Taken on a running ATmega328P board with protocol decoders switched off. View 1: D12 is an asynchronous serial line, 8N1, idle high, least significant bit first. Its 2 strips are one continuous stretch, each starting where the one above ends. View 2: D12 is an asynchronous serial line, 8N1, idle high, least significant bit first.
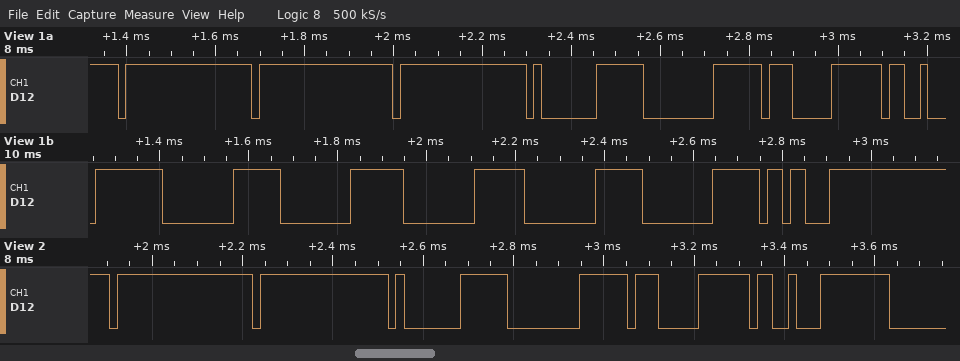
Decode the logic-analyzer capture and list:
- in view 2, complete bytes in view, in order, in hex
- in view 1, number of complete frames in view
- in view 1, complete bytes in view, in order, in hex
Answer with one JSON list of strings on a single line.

["FF FF 01 00 07 13", "13", "0xFF 0xFF 0xFF 0x01 0x00 0x07 0x13 0x00 0x00 0x00 0x00 0x00 0x1B"]
